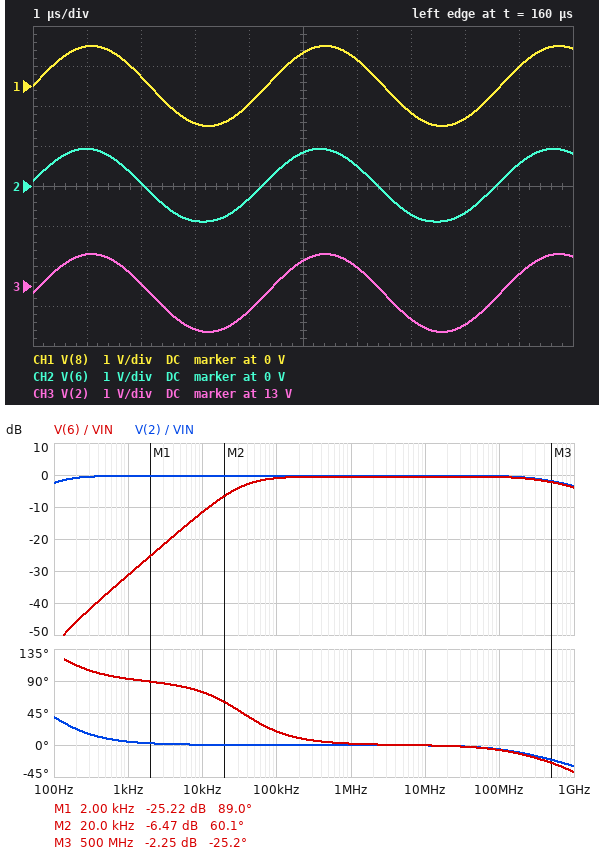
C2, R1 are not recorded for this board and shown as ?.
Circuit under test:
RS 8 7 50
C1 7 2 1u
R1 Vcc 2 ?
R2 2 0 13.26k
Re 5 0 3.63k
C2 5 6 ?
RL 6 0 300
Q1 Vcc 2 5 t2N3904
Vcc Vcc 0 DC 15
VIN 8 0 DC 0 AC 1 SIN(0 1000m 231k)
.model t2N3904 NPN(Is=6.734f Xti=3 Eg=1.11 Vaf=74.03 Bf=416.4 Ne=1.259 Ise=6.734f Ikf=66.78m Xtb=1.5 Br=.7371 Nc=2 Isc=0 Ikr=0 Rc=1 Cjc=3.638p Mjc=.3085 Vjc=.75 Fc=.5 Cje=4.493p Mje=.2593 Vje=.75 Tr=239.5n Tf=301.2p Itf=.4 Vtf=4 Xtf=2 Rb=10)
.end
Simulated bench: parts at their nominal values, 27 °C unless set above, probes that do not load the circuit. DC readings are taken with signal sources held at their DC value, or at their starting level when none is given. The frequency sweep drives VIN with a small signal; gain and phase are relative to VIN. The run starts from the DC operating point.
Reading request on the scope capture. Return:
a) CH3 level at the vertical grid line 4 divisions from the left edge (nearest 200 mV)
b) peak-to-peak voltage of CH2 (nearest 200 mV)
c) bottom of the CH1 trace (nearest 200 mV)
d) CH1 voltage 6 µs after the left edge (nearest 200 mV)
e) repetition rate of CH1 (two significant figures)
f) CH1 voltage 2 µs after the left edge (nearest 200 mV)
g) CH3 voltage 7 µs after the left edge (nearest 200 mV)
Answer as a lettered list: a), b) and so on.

a) 12.4 V
b) 1.8 V
c) -1.0 V
d) 600 mV
e) 230 kHz
f) 200 mV
g) 12.2 V
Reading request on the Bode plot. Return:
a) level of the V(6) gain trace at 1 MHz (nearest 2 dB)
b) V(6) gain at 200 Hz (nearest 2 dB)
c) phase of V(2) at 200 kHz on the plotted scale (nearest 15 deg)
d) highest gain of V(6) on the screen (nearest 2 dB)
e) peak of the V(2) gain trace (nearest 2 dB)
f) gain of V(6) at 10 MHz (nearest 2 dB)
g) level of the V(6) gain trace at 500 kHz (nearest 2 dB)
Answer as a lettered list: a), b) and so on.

a) 0 dB
b) -46 dB
c) 0 deg
d) 0 dB
e) 0 dB
f) 0 dB
g) 0 dB
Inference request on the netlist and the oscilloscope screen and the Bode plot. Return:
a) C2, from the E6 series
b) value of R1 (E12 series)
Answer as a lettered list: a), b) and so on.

a) 15 nF
b) 2.2 kΩ
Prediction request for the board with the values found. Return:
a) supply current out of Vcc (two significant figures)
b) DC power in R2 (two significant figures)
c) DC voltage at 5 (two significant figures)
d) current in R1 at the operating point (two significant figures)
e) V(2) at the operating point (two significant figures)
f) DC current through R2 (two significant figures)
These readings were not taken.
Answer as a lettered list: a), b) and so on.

a) 4.3 mA
b) 12 mW
c) 12 V
d) 990 µA
e) 13 V
f) 970 µA
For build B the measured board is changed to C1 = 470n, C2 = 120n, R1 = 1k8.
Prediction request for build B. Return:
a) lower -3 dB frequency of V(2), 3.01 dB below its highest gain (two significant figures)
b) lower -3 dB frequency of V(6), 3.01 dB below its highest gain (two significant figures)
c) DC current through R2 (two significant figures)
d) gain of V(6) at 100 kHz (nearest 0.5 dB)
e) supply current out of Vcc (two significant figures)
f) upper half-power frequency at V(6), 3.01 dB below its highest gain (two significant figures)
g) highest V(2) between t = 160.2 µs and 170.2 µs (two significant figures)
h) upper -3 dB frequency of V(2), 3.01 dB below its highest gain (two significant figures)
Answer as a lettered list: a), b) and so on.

a) 210 Hz
b) 4.3 kHz
c) 990 µA
d) -0.5 dB
e) 4.4 mA
f) 830 MHz
g) 14 V
h) 880 MHz
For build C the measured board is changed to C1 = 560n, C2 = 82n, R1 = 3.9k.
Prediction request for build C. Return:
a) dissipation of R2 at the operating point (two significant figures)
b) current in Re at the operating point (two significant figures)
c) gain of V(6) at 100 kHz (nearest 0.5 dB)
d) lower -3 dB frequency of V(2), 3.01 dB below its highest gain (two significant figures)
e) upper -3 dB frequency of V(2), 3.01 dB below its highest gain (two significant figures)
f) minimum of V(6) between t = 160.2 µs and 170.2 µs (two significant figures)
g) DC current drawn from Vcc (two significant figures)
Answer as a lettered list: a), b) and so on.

a) 10 mW
b) 3.0 mA
c) -0.5 dB
d) 93 Hz
e) 1.0 GHz
f) -830 mV
g) 3.9 mA
